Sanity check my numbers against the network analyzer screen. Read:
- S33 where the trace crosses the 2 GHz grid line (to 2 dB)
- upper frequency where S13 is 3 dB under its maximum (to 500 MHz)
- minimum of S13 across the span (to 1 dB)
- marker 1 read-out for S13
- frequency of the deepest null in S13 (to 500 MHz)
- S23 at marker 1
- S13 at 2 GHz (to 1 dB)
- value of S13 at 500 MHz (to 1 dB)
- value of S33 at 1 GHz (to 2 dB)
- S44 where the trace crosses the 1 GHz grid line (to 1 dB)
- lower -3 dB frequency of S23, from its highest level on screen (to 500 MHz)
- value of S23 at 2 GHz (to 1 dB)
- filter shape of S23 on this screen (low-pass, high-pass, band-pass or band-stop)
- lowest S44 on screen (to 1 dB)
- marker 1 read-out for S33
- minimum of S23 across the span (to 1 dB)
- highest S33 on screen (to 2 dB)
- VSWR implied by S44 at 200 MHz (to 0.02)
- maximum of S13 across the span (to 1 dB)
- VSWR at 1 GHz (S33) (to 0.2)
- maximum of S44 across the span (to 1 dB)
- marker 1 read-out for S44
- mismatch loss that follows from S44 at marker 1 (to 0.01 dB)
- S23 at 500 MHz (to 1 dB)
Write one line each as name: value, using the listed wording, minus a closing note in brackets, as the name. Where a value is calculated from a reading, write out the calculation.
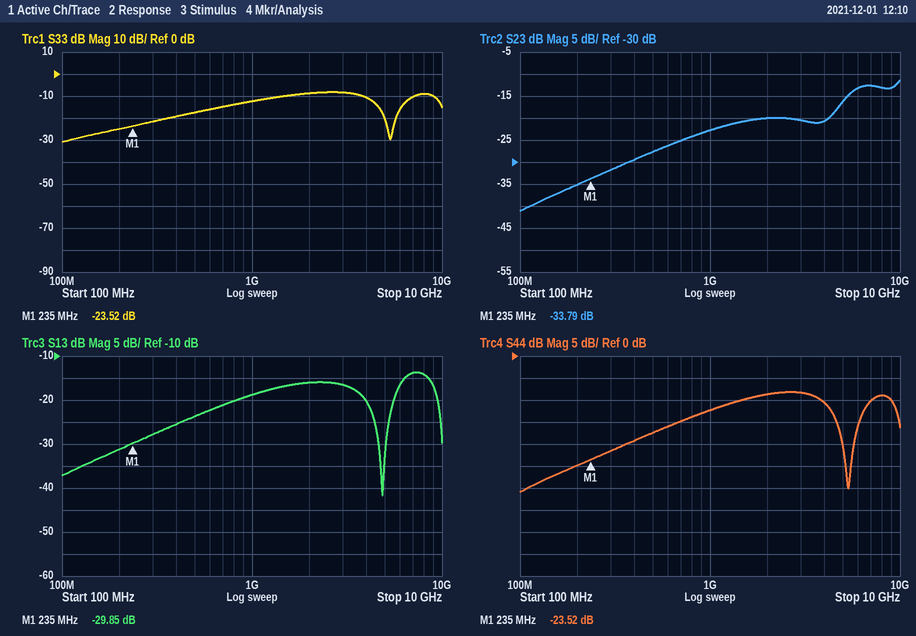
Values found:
S33 where the trace crosses the 2 GHz grid line: -8 dB
upper frequency where S13 is 3 dB under its maximum: 9.0 GHz
minimum of S13 across the span: -42 dB
marker 1 read-out for S13: -29.85 dB
frequency of the deepest null in S13: 5.0 GHz
S23 at marker 1: -33.79 dB
S13 at 2 GHz: -16 dB
value of S13 at 500 MHz: -24 dB
value of S33 at 1 GHz: -12 dB
S44 where the trace crosses the 1 GHz grid line: -12 dB
lower -3 dB frequency of S23, from its highest level on screen: 5.5 GHz
value of S23 at 2 GHz: -20 dB
filter shape of S23 on this screen: high-pass
lowest S44 on screen: -31 dB
marker 1 read-out for S33: -23.52 dB
minimum of S23 across the span: -41 dB
highest S33 on screen: -8 dB
VSWR implied by S44 at 200 MHz: |Γ| = 10^(-25/20) = 0.0562; VSWR = (1 + 0.0562)/(1 − 0.0562) ≈ 1.12
maximum of S13 across the span: -14 dB
VSWR at 1 GHz (S33): |Γ| = 10^(-12/20) = 0.2512; VSWR = (1 + 0.2512)/(1 − 0.2512) ≈ 1.67, so 1.6 to the nearest 0.2
maximum of S44 across the span: -8 dB
marker 1 read-out for S44: -23.52 dB
mismatch loss that follows from S44 at marker 1: −10 log10(1 − 10^(-23.52/10)) ≈ 0.02 dB
S23 at 500 MHz: -28 dB
